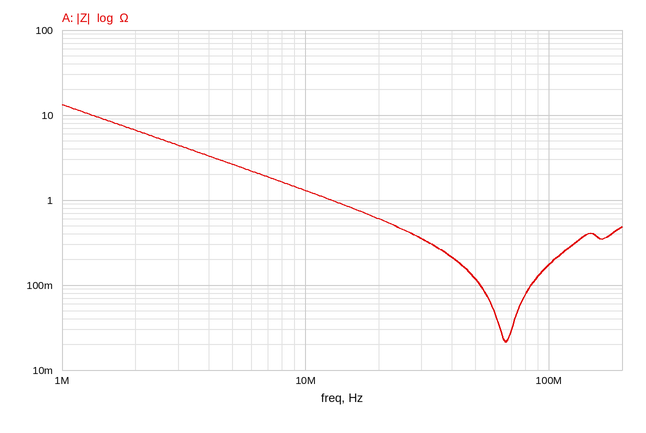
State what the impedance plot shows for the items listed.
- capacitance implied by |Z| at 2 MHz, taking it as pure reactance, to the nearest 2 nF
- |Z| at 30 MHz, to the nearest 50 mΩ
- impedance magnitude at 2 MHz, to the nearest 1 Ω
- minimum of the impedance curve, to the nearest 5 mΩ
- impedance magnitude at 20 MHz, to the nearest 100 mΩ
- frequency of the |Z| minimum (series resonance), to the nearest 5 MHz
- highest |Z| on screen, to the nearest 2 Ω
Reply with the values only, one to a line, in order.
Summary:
12 nF
350 mΩ
7 Ω
20 mΩ
600 mΩ
65 MHz
14 Ω
